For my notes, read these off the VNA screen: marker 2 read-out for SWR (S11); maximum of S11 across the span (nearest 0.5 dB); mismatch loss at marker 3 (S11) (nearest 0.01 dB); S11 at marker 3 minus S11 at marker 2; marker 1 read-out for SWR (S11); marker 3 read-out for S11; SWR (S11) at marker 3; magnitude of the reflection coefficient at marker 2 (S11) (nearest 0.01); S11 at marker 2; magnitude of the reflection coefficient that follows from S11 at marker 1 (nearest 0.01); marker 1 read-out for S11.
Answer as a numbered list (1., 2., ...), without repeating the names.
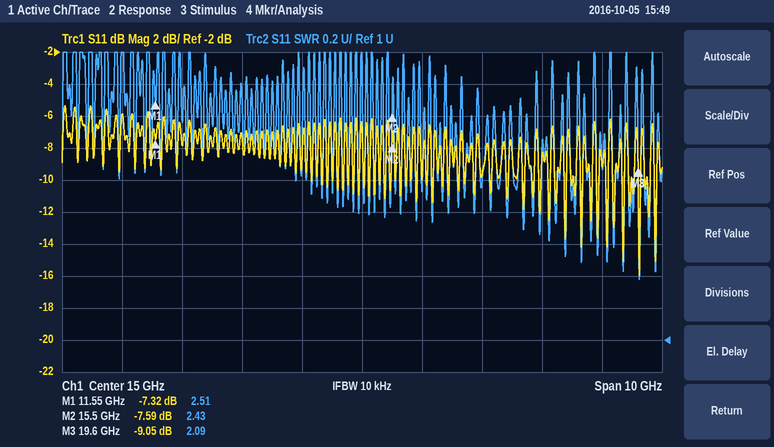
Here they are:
1. 2.43
2. -5.5 dB
3. 0.58 dB
4. -1.46 dB
5. 2.51
6. -9.05 dB
7. 2.09
8. 0.42
9. -7.59 dB
10. 0.43
11. -7.32 dB
